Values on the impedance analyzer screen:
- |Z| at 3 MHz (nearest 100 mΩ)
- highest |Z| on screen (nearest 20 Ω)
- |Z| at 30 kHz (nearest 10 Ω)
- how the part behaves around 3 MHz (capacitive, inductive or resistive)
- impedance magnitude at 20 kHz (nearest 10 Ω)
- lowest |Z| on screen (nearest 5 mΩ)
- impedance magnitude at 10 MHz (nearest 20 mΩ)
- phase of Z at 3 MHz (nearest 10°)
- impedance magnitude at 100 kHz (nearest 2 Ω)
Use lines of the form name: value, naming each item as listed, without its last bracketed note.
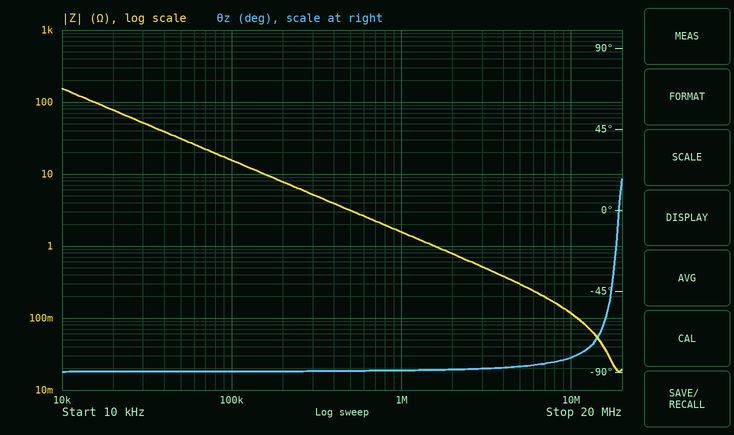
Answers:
|Z| at 3 MHz: 500 mΩ
highest |Z| on screen: 160 Ω
|Z| at 30 kHz: 50 Ω
how the part behaves around 3 MHz: capacitive
impedance magnitude at 20 kHz: 80 Ω
lowest |Z| on screen: 20 mΩ
impedance magnitude at 10 MHz: 120 mΩ
phase of Z at 3 MHz: -90°
impedance magnitude at 100 kHz: 16 Ω
